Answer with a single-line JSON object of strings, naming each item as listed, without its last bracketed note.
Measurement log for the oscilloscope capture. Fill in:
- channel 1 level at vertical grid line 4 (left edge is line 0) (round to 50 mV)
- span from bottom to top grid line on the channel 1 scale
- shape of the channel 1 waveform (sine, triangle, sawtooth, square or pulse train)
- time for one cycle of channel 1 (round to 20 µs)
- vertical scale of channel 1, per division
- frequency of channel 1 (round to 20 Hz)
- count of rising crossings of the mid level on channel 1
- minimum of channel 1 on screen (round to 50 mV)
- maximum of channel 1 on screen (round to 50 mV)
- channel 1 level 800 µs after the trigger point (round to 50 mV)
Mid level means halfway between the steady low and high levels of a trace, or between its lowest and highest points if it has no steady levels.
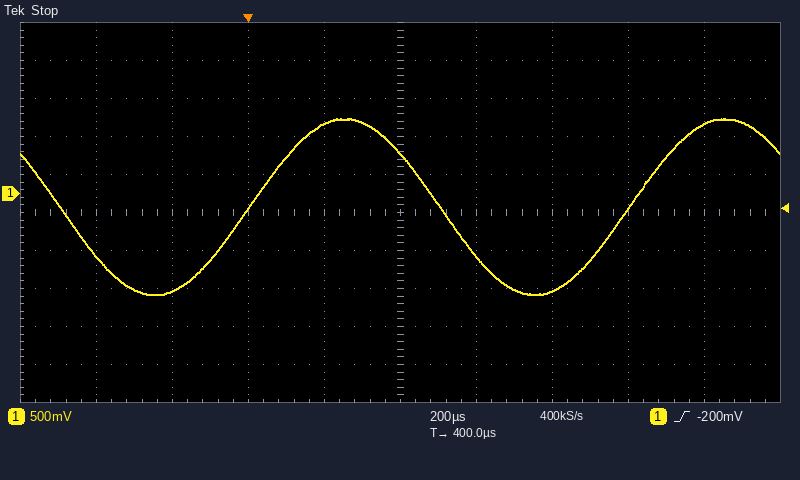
{"channel 1 level at vertical grid line 4 (left edge is line 0)": "900 mV", "span from bottom to top grid line on the channel 1 scale": "5 V", "shape of the channel 1 waveform": "sine", "time for one cycle of channel 1": "1.00 ms", "vertical scale of channel 1, per division": "500 mV", "frequency of channel 1": "1.00 kHz", "count of rising crossings of the mid level on channel 1": "2", "minimum of channel 1 on screen": "-1.35 V", "maximum of channel 1 on screen": "1.00 V", "channel 1 level 800 µs after the trigger point": "-1.30 V"}
